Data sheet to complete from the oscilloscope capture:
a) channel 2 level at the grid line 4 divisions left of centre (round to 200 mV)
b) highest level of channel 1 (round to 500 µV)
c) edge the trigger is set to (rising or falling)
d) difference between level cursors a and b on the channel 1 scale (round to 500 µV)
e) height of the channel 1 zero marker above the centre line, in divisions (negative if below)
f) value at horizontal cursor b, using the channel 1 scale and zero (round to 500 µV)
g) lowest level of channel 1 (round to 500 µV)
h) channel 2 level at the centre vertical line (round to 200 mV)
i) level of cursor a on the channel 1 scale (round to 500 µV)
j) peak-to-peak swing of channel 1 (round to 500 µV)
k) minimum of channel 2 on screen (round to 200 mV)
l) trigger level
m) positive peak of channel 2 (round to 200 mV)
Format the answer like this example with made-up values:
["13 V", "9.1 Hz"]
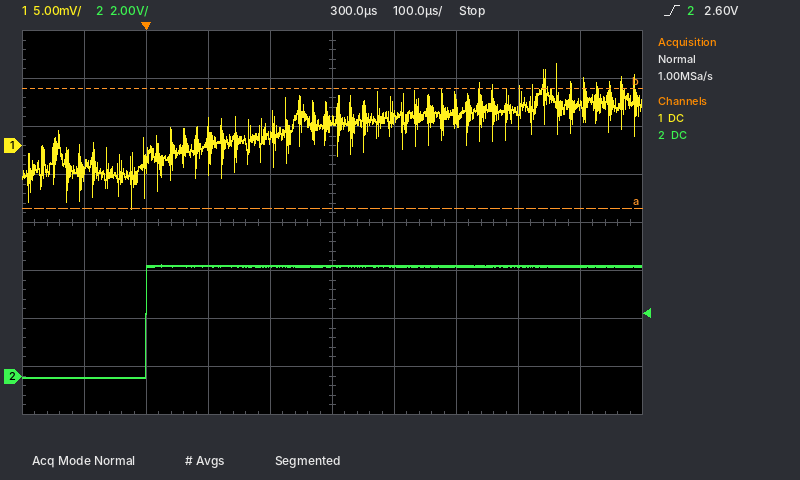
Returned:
["0.0 V", "8.5 mV", "rising", "12.5 mV", "+1.6 div", "6.0 mV", "-6.5 mV", "4.6 V", "-6.5 mV", "15.0 mV", "0.0 V", "2.60 V", "4.6 V"]
